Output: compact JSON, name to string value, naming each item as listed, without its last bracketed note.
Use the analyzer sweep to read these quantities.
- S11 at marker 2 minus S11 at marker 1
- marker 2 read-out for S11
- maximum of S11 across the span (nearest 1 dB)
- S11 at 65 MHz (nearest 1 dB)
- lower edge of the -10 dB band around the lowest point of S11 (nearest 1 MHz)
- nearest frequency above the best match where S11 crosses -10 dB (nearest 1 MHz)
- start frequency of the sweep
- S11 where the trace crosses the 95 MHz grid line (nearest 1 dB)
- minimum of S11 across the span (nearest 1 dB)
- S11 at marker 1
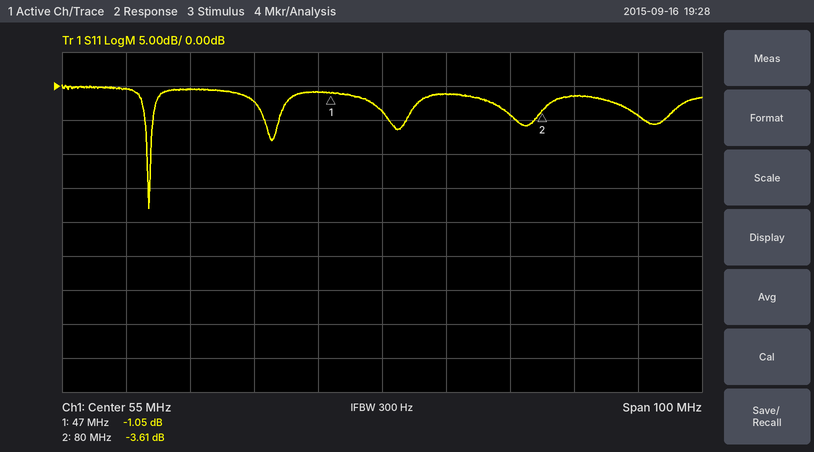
{"S11 at marker 2 minus S11 at marker 1": "-2.56 dB", "marker 2 read-out for S11": "-3.61 dB", "maximum of S11 across the span": "0 dB", "S11 at 65 MHz": "-1 dB", "lower edge of the -10 dB band around the lowest point of S11": "18 MHz", "nearest frequency above the best match where S11 crosses -10 dB": "19 MHz", "start frequency of the sweep": "5 MHz", "S11 where the trace crosses the 95 MHz grid line": "-4 dB", "minimum of S11 across the span": "-18 dB", "S11 at marker 1": "-1.05 dB"}
